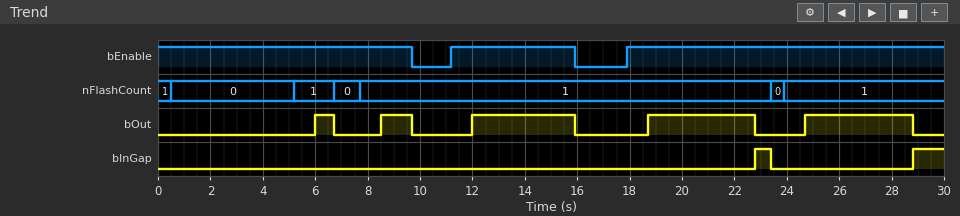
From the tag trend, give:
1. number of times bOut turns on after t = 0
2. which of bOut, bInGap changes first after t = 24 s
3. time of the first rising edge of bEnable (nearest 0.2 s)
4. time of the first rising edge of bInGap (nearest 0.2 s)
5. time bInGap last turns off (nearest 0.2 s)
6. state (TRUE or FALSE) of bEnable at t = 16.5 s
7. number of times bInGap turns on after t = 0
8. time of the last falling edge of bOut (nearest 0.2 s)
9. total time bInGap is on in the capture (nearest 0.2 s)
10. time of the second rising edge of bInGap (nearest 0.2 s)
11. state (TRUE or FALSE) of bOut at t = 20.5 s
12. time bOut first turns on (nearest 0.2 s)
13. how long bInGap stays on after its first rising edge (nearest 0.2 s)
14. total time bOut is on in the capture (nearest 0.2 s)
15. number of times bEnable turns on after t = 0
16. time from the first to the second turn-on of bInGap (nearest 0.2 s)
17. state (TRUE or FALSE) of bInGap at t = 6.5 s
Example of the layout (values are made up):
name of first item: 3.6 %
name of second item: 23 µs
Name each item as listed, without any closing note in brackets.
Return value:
number of times bOut turns on after t = 0: 5
which of bOut, bInGap changes first after t = 24 s: bOut
time of the first rising edge of bEnable: 11.2 s
time of the first rising edge of bInGap: 22.8 s
time bInGap last turns off: 23.4 s
state (TRUE or FALSE) of bEnable at t = 16.5 s: FALSE
number of times bInGap turns on after t = 0: 2
time of the last falling edge of bOut: 28.8 s
total time bInGap is on in the capture: 1.8 s
time of the second rising edge of bInGap: 28.8 s
state (TRUE or FALSE) of bOut at t = 20.5 s: TRUE
time bOut first turns on: 6.0 s
how long bInGap stays on after its first rising edge: 0.6 s
total time bOut is on in the capture: 14.0 s
number of times bEnable turns on after t = 0: 2
time from the first to the second turn-on of bInGap: 6.0 s
state (TRUE or FALSE) of bInGap at t = 6.5 s: FALSE
